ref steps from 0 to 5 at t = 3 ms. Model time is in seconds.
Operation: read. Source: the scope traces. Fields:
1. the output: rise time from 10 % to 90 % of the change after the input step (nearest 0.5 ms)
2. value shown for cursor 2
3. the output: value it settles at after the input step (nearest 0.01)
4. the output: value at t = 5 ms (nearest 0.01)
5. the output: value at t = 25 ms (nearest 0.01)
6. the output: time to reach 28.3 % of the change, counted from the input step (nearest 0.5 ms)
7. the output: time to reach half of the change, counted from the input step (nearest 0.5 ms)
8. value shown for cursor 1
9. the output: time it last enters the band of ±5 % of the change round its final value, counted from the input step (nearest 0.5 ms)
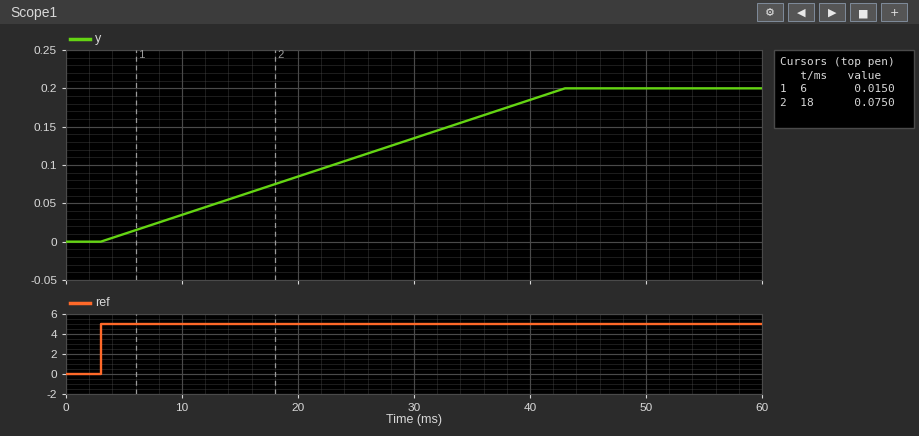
32.0 ms
0.0750
0.20
0.01
0.11
11.5 ms
20.0 ms
0.0150
38.0 ms
